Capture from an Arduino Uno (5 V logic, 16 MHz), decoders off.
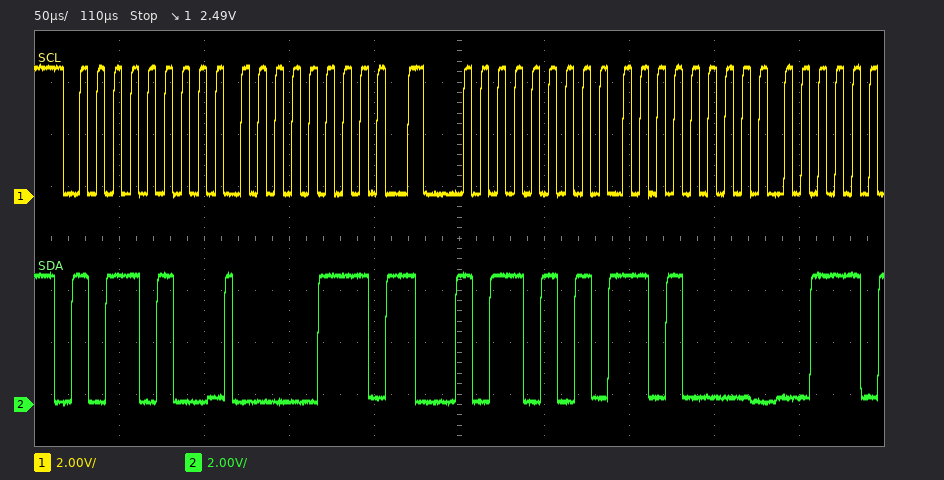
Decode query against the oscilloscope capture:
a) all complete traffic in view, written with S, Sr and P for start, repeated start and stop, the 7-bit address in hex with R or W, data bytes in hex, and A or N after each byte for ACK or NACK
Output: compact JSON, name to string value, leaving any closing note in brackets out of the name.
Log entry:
{"all complete traffic in view, written with S, Sr and P for start, repeated start and stop, the 7-bit address in hex with R or W, data bytes in hex, and A or N after each byte for ACK or NACK": "S 5AW A 07 A Sr 5AR A D0 A"}
